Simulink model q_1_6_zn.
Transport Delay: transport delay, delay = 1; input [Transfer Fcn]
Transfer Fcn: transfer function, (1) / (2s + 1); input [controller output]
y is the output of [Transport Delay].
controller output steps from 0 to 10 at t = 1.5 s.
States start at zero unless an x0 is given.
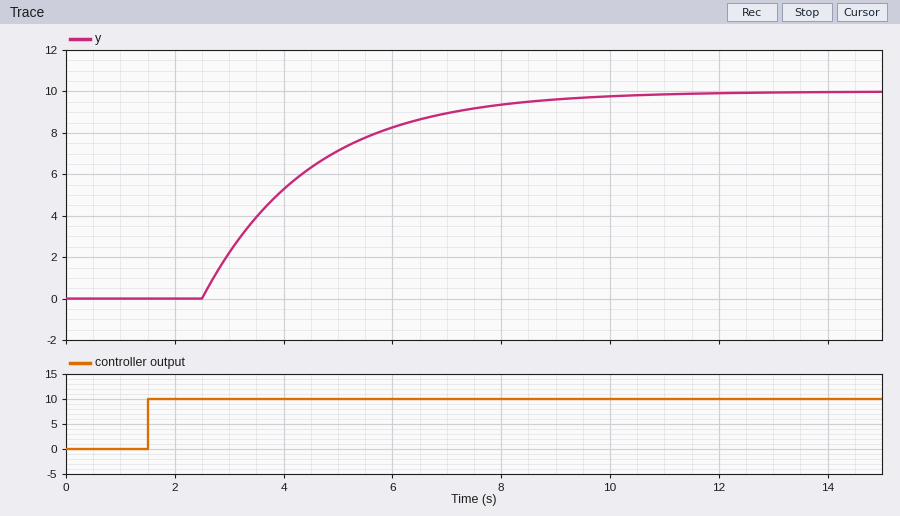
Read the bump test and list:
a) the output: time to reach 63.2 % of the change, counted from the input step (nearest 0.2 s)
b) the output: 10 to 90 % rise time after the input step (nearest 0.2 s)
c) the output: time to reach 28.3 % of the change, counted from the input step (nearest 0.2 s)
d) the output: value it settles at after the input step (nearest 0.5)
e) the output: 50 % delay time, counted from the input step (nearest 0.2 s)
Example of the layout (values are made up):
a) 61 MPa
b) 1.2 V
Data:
a) 3.0 s
b) 4.4 s
c) 1.6 s
d) 10.0
e) 2.4 s
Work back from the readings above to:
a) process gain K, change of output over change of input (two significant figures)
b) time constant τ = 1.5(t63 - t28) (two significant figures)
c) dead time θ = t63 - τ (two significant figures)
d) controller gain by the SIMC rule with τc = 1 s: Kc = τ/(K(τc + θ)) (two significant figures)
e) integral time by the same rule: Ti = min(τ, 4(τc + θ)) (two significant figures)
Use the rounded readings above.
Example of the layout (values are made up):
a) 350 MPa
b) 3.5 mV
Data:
a) 1.0
b) 2.1 s
c) 0.90 s
d) 1.1
e) 2.1 s
